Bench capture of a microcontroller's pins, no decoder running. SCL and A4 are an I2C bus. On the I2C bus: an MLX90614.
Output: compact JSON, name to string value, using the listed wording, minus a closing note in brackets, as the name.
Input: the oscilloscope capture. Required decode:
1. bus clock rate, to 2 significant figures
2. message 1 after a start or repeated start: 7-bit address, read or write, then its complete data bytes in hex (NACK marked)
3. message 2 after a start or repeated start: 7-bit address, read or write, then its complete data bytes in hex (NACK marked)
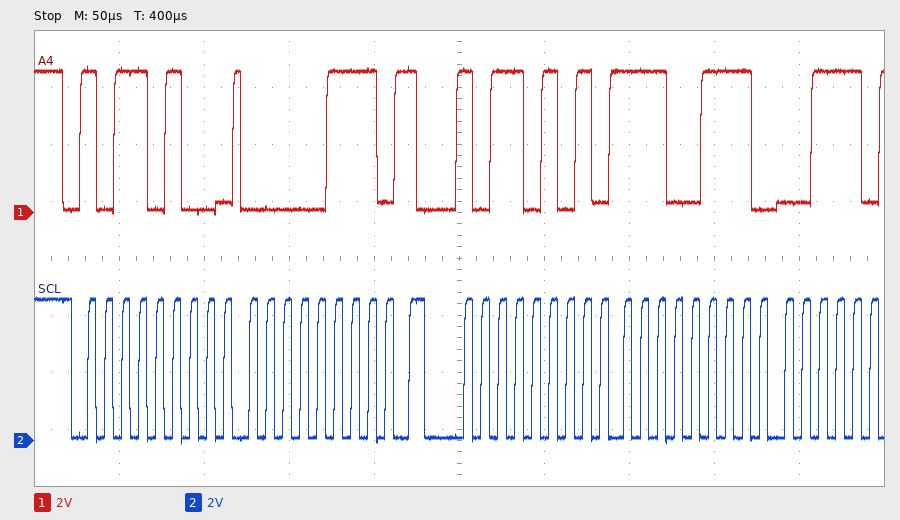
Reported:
{"bus clock rate, to 2 significant figures": "100 kHz", "message 1 after a start or repeated start: 7-bit address, read or write, then its complete data bytes in hex": "0x5A write: 07", "message 2 after a start or repeated start: 7-bit address, read or write, then its complete data bytes in hex": "0x5A read: E7"}
